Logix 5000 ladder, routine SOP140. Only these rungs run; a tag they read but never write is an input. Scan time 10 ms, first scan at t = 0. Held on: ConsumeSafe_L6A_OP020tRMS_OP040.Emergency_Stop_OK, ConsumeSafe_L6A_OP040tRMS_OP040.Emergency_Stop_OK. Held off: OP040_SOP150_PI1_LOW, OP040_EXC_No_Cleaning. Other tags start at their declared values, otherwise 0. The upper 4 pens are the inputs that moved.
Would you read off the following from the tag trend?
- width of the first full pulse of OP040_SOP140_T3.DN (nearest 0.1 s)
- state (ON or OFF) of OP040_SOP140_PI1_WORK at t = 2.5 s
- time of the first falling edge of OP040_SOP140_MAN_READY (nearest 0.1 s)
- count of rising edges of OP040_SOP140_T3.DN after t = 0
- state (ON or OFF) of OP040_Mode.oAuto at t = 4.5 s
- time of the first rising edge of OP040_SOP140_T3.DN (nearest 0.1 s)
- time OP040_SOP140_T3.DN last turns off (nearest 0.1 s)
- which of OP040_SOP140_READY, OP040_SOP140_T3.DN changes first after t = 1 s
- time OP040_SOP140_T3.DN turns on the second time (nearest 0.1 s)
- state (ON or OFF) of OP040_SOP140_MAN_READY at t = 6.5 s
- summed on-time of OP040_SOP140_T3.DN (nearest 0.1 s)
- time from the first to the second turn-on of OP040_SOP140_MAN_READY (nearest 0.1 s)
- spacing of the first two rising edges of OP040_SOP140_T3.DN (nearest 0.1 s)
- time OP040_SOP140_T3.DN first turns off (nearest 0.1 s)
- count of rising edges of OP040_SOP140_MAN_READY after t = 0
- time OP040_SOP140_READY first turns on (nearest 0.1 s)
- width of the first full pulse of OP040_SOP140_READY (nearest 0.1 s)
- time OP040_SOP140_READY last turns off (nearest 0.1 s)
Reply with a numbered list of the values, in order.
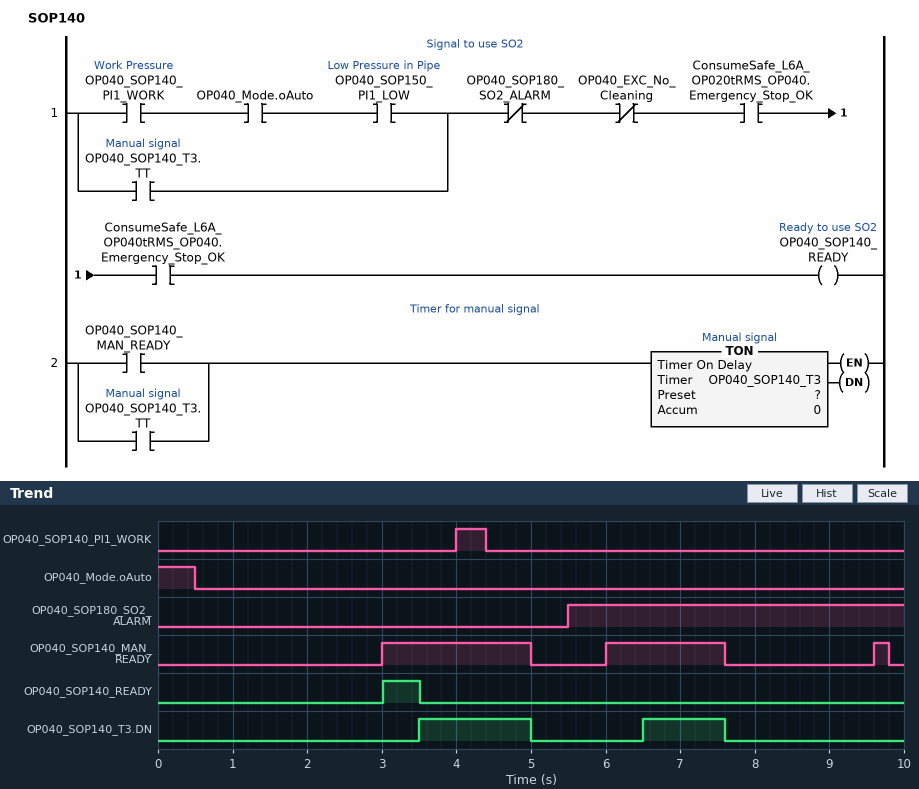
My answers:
1. 1.5 s
2. OFF
3. 5.0 s
4. 2
5. OFF
6. 3.5 s
7. 7.6 s
8. OP040_SOP140_READY
9. 6.5 s
10. ON
11. 2.6 s
12. 3.0 s
13. 3.0 s
14. 5.0 s
15. 3
16. 3.0 s
17. 0.5 s
18. 3.5 s
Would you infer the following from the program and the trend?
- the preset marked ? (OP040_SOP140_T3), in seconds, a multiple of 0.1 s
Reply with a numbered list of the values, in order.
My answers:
1. 0.5 s
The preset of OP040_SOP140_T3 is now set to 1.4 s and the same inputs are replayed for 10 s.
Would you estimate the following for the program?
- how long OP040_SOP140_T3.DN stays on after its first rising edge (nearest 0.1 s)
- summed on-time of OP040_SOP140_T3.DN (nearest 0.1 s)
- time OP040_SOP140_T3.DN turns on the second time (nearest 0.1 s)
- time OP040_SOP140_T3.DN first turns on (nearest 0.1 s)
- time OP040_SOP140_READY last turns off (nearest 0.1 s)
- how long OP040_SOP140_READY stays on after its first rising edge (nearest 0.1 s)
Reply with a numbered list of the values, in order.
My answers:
1. 0.6 s
2. 0.8 s
3. 7.4 s
4. 4.4 s
5. 4.4 s
6. 1.4 s
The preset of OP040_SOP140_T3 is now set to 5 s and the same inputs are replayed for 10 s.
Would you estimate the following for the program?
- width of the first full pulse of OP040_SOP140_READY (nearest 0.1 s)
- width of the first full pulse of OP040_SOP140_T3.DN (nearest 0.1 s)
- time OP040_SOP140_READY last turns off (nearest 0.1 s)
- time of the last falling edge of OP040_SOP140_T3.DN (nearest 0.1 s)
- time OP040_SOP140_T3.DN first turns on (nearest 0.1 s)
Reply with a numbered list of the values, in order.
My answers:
1. 2.5 s
2. 0.0 s
3. 5.5 s
4. 8.0 s
5. 8.0 s
